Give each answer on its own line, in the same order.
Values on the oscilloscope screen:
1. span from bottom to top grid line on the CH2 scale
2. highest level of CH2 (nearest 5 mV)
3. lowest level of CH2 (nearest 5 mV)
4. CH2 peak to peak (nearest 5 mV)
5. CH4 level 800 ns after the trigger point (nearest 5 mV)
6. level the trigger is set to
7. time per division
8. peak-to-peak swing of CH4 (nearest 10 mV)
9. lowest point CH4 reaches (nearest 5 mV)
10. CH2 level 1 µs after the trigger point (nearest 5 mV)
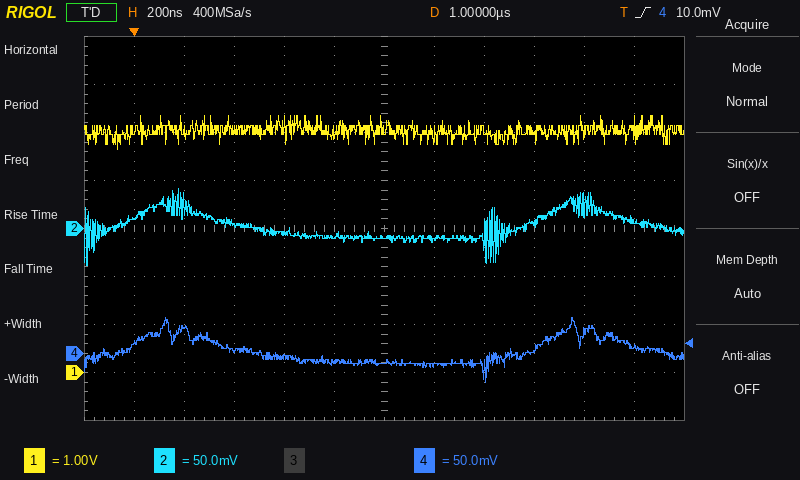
400 mV
40 mV
-40 mV
80 mV
-10 mV
10.0 mV
200 ns
70 mV
-30 mV
-10 mV
